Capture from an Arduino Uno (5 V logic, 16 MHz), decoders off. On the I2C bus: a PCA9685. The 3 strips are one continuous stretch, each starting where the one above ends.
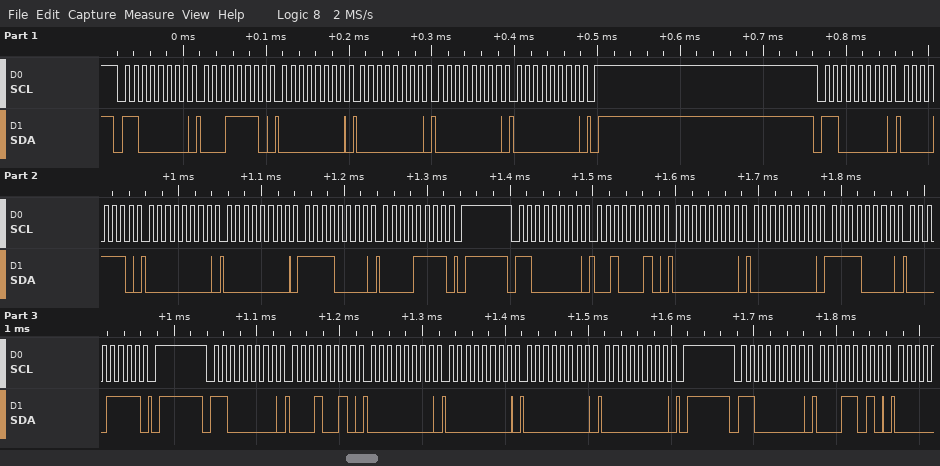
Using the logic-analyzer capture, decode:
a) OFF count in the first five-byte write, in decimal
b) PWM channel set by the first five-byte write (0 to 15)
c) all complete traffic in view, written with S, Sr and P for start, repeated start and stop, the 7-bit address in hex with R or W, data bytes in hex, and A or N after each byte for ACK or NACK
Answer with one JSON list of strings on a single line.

["0", "6", "S 60W A 1E A 00 A 00 A 00 A 00 A P S 60W A 0E A 00 A 00 A F0 A 0F A P S 60W A 22 A 00 A 00 A F0 A 0F A P S 60W A 12 A 00 A 00 A 00 A 00 A P S 60W A 1A A"]
